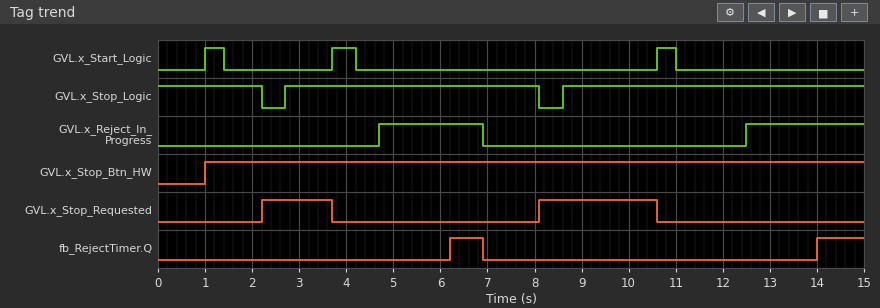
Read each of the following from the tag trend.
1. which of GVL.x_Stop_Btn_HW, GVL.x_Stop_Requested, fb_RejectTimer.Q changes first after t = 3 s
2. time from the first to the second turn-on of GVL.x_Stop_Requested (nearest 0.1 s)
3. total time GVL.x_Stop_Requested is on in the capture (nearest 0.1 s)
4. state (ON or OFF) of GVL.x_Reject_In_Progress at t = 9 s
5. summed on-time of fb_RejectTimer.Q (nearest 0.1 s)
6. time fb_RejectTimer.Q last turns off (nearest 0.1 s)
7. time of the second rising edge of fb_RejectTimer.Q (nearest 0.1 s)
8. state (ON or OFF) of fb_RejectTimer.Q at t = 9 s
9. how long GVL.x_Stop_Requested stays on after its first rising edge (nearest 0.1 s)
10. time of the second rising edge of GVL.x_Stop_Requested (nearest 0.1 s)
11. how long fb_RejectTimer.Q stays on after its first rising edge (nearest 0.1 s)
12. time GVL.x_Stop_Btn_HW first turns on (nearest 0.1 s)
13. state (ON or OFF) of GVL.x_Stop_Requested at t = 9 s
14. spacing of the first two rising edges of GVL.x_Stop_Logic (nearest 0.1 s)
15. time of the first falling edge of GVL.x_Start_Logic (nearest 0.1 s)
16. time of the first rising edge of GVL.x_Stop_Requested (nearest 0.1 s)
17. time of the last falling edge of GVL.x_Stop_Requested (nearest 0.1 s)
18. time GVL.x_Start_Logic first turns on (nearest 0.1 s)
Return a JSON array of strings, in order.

["GVL.x_Stop_Requested", "5.9 s", "4.0 s", "OFF", "1.7 s", "6.9 s", "14.0 s", "OFF", "1.5 s", "8.1 s", "0.7 s", "1.0 s", "ON", "5.9 s", "1.4 s", "2.2 s", "10.6 s", "1.0 s"]
